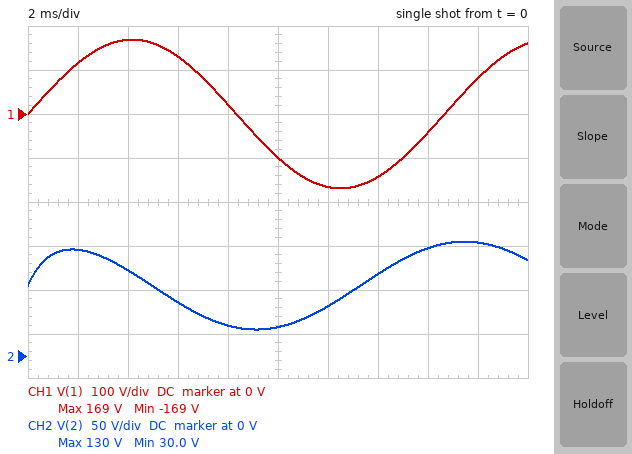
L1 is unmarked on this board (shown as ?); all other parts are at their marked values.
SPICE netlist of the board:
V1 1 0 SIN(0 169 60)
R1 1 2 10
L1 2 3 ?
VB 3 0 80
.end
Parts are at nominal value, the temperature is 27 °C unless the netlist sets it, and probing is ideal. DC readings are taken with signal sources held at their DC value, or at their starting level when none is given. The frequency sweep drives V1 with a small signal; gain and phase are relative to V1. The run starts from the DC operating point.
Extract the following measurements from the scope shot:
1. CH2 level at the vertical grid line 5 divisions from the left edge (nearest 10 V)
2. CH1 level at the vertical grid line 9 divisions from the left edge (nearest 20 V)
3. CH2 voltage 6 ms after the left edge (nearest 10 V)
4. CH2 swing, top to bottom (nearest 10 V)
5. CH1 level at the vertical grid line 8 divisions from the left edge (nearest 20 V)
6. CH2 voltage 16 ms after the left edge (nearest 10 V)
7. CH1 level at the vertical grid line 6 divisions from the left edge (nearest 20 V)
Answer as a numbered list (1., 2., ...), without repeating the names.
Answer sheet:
1. 30 V
2. 80 V
3. 60 V
4. 100 V
5. -40 V
6. 120 V
7. -160 V
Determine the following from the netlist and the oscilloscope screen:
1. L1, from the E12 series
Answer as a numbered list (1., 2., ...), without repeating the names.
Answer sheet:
1. 8.2 mH
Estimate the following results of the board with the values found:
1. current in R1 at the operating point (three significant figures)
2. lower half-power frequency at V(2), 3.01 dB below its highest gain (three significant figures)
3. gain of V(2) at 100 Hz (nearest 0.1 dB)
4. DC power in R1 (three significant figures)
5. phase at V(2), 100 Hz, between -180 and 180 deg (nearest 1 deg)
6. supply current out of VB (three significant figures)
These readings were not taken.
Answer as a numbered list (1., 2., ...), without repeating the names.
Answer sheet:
1. 8.00 A
2. 194 Hz
3. -6.8 dB
4. 640 W
5. 63 deg
6. 8.00 A
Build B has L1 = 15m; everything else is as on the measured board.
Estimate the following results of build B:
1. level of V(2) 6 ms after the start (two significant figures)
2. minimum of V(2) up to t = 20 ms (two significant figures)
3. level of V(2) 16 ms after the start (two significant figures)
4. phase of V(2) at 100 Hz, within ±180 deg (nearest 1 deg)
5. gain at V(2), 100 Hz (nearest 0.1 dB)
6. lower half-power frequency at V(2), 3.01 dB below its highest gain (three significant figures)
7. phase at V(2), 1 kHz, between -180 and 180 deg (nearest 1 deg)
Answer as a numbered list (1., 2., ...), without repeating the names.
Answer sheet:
1. 64 V
2. -3.3 V
3. 140 V
4. 47 deg
5. -3.3 dB
6. 106 Hz
7. 6 deg
